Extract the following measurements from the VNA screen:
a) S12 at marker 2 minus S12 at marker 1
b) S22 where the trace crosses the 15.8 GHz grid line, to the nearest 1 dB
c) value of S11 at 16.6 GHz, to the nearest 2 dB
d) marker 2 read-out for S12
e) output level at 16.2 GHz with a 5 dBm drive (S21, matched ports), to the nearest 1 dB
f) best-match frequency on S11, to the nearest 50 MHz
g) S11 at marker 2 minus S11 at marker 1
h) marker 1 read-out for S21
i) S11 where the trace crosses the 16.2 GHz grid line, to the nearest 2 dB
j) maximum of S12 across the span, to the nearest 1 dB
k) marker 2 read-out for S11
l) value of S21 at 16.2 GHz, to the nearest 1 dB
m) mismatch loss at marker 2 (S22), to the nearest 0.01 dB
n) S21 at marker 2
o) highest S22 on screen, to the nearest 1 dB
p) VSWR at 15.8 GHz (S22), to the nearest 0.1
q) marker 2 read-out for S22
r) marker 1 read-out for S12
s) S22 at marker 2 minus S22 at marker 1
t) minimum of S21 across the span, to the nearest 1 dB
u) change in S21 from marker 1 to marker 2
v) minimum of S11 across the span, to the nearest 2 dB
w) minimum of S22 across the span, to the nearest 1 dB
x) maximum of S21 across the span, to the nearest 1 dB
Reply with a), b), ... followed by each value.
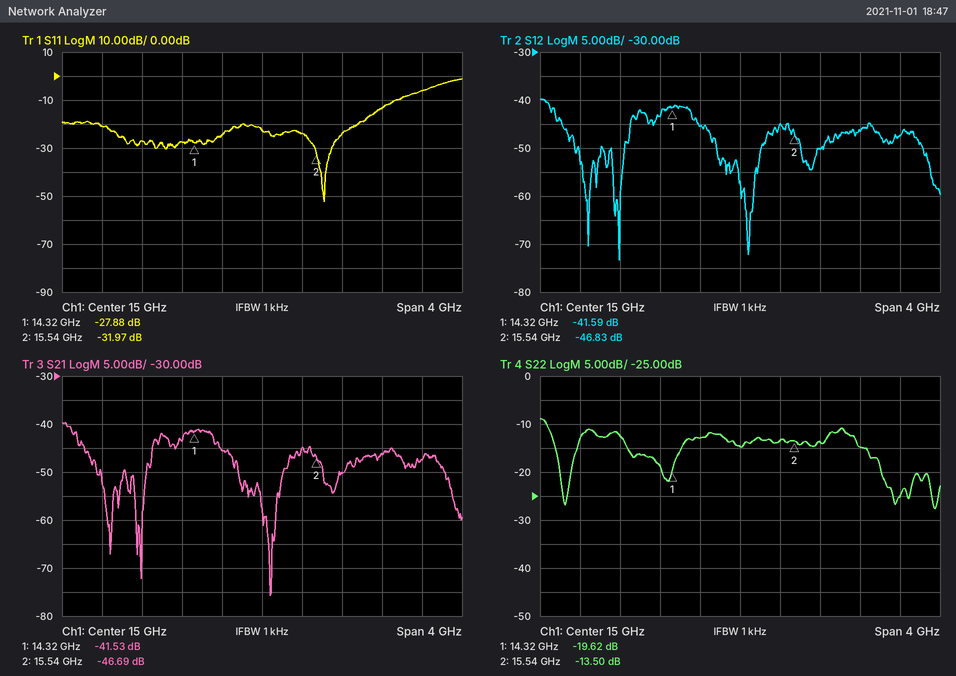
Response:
a) -5.24 dB
b) -14 dB
c) -6 dB
d) -46.83 dB
e) -41 dBm
f) 15.60 GHz
g) -4.09 dB
h) -41.53 dB
i) -14 dB
j) -40 dB
k) -31.97 dB
l) -46 dB
m) 0.20 dB
n) -46.69 dB
o) -9 dB
p) 1.5
q) -13.50 dB
r) -41.59 dB
s) 6.12 dB
t) -76 dB
u) -5.16 dB
v) -52 dB
w) -28 dB
x) -40 dB
